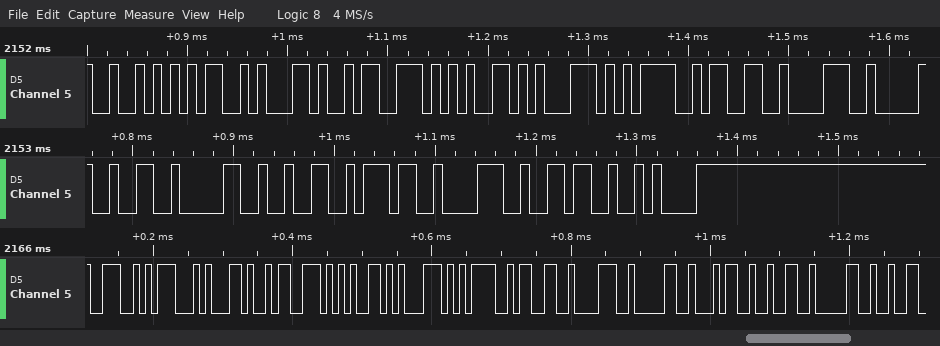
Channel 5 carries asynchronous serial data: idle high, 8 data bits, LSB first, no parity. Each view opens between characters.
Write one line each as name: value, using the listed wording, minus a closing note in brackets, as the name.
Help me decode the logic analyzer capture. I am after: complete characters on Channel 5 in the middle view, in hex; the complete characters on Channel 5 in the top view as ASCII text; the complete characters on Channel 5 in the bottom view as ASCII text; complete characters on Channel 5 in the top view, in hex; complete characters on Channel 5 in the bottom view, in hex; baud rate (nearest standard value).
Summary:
complete characters on Channel 5 in the middle view, in hex: 32, 30, 32, 37, 38, 36, 0A
the complete characters on Channel 5 in the top view as ASCII text: "RM,seq=38"
the complete characters on Channel 5 in the bottom view as ASCII text: "NG,seq=380420"
complete characters on Channel 5 in the top view, in hex: 52, 4D, 2C, 73, 65, 71, 3D, 33, 38
complete characters on Channel 5 in the bottom view, in hex: 4E, 47, 2C, 73, 65, 71, 3D, 33, 38, 30, 34, 32, 30
baud rate: 115200 baud
